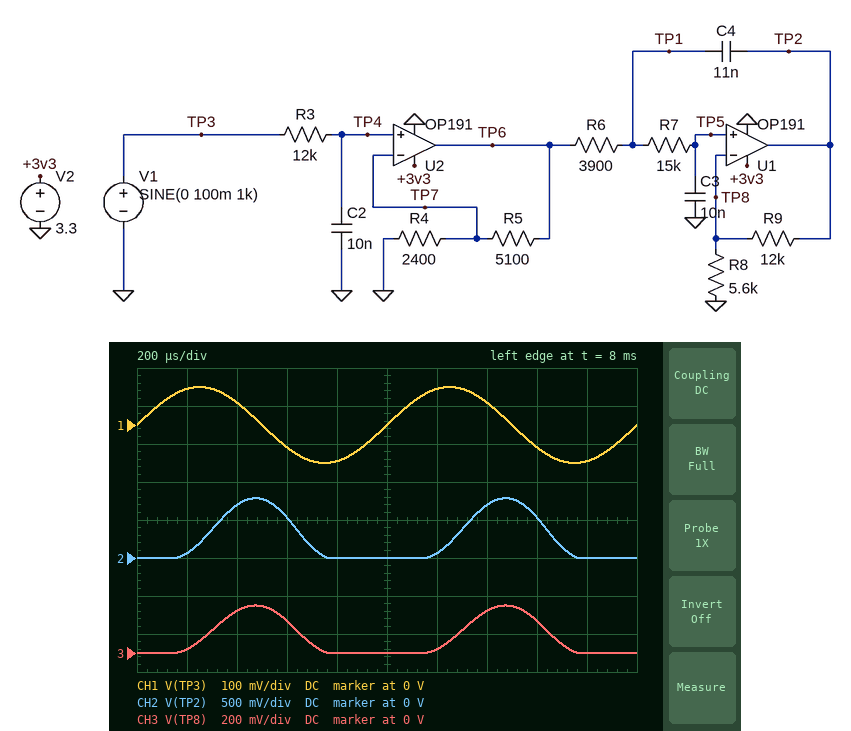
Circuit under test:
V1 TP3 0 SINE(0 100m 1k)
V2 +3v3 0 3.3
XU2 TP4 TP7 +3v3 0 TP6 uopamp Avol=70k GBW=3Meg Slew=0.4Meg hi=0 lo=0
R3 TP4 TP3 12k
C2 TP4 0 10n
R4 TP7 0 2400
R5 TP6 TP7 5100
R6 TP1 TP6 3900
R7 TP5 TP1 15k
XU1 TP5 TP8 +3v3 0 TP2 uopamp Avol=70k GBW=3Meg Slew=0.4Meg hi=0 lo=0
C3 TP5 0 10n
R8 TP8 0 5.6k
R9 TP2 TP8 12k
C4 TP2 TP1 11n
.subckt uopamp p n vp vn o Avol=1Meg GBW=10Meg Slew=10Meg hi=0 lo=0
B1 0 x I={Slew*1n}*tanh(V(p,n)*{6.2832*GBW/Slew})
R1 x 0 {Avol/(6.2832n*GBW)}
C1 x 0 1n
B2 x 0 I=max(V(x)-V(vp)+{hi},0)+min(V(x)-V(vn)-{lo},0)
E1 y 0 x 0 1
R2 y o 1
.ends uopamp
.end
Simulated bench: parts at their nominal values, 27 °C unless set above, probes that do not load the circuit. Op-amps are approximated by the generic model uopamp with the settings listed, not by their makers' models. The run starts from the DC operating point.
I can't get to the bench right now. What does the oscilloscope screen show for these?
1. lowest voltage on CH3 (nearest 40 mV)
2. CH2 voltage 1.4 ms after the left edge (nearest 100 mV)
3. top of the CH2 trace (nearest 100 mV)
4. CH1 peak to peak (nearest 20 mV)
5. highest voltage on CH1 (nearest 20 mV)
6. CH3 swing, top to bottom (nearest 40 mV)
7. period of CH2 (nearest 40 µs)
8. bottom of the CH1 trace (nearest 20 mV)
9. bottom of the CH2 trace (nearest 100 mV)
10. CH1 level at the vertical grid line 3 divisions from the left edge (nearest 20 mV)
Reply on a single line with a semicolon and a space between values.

0 V; 700 mV; 800 mV; 200 mV; 100 mV; 240 mV; 1.00 ms; -100 mV; 0 V; -60 mV
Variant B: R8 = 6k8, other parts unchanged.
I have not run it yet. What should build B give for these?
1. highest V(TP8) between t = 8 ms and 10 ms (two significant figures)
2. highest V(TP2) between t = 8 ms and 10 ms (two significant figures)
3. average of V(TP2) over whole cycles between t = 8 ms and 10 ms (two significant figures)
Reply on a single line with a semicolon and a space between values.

240 mV; 650 mV; 220 mV
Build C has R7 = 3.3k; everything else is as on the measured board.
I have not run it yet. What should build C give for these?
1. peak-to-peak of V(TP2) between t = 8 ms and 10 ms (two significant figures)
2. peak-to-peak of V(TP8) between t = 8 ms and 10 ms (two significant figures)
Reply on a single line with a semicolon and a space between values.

2.1 V; 680 mV
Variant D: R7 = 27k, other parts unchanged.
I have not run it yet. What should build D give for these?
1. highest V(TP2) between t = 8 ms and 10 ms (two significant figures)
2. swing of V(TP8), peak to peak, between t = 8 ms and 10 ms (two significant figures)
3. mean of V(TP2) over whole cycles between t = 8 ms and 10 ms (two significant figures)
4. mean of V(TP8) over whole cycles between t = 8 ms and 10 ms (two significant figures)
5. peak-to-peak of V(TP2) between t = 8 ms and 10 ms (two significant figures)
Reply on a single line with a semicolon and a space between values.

570 mV; 180 mV; 250 mV; 79 mV; 550 mV
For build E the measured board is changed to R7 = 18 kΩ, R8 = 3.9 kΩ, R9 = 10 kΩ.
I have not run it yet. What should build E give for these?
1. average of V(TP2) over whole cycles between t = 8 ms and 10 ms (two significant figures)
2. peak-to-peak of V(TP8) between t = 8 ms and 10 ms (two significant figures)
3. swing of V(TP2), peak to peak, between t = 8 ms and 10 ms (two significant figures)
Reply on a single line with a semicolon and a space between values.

290 mV; 240 mV; 870 mV
